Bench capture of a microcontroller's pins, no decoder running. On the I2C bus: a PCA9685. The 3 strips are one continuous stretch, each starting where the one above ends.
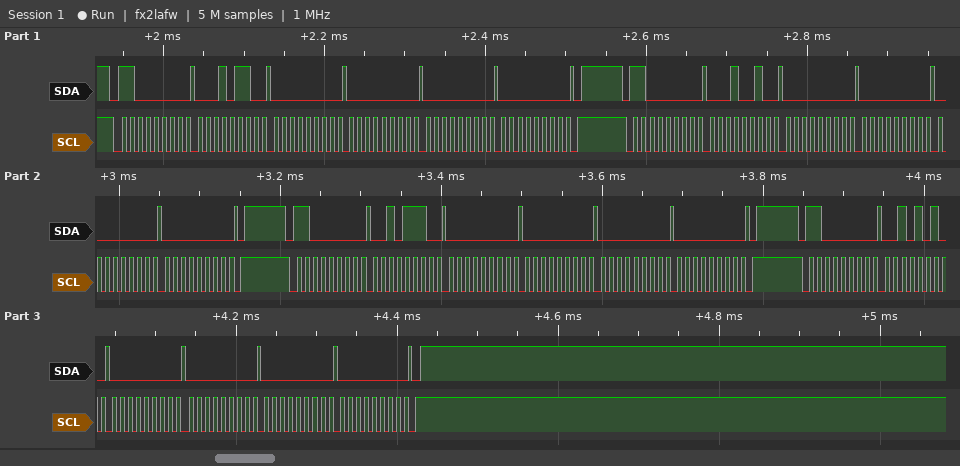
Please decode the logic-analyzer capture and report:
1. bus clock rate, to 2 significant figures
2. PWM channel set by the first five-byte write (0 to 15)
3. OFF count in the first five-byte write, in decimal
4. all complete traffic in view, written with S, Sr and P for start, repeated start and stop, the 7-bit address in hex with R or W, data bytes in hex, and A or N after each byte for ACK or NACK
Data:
100 kHz
4
0
S 60W A 16 A 00 A 00 A 00 A 00 A P S 60W A 12 A 00 A 00 A 00 A 00 A P S 60W A 2E A 00 A 00 A 00 A 00 A P S 60W A 2A A 00 A 00 A 00 A 00 A P
